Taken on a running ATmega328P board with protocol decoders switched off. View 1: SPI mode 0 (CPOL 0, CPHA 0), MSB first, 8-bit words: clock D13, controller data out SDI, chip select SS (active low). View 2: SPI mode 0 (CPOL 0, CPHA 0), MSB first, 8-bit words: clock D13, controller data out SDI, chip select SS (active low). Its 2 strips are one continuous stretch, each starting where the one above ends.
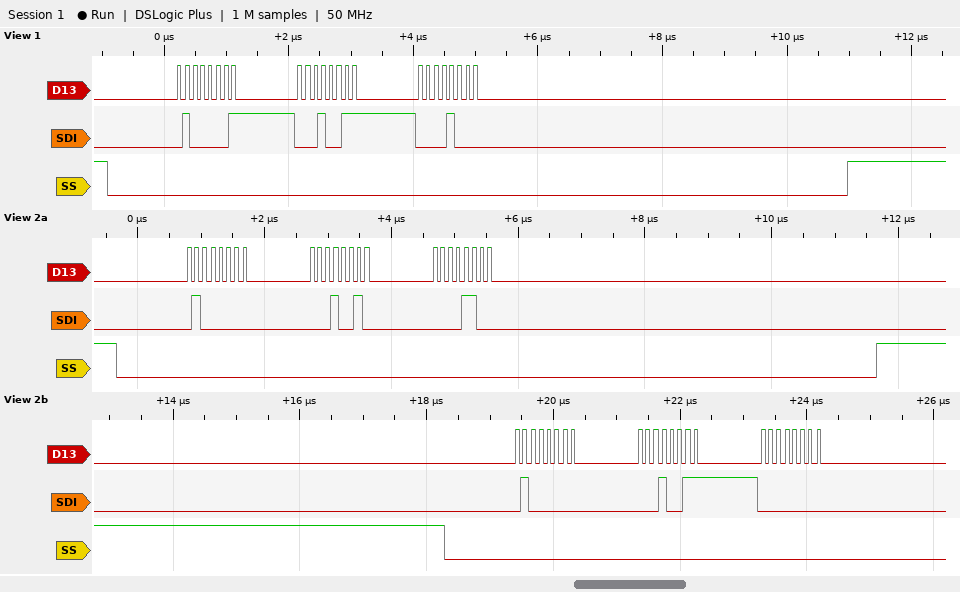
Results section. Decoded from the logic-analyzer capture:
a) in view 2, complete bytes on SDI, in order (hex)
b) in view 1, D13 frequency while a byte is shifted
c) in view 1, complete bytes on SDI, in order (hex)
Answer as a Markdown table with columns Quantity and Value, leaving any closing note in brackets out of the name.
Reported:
| Quantity | Value |
|---|---|
| in view 2, complete bytes on SDI, in order | 40 12 0C 40 13 00 |
| in view 1, D13 frequency while a byte is shifted | 8 MHz |
| in view 1, complete bytes on SDI, in order | 41 13 08 |
